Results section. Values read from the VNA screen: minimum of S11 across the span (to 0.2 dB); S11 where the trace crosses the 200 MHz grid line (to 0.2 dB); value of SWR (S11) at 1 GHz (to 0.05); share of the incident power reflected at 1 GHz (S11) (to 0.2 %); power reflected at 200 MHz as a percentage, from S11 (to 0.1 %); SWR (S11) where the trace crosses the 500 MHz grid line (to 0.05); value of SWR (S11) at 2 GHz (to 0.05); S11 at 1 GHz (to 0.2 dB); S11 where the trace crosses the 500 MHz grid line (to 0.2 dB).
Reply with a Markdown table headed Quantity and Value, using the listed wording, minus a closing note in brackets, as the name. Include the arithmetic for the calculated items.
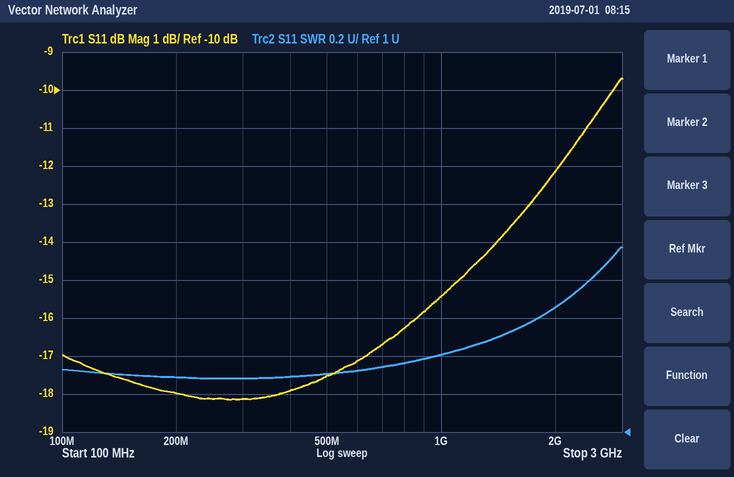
| Quantity | Value |
|---|---|
| minimum of S11 across the span | -18.2 dB |
| S11 where the trace crosses the 200 MHz grid line | -18.0 dB |
| value of SWR (S11) at 1 GHz | 1.40 |
| share of the incident power reflected at 1 GHz (S11) | 10^(-15.4/10) ≈ 2.88 %, so 2.8 % to the nearest 0.2 % |
| power reflected at 200 MHz as a percentage, from S11 | 10^(-18/10) ≈ 1.6 % |
| SWR (S11) where the trace crosses the 500 MHz grid line | 1.30 |
| value of SWR (S11) at 2 GHz | 1.65 |
| S11 at 1 GHz | -15.4 dB |
| S11 where the trace crosses the 500 MHz grid line | -17.6 dB |
